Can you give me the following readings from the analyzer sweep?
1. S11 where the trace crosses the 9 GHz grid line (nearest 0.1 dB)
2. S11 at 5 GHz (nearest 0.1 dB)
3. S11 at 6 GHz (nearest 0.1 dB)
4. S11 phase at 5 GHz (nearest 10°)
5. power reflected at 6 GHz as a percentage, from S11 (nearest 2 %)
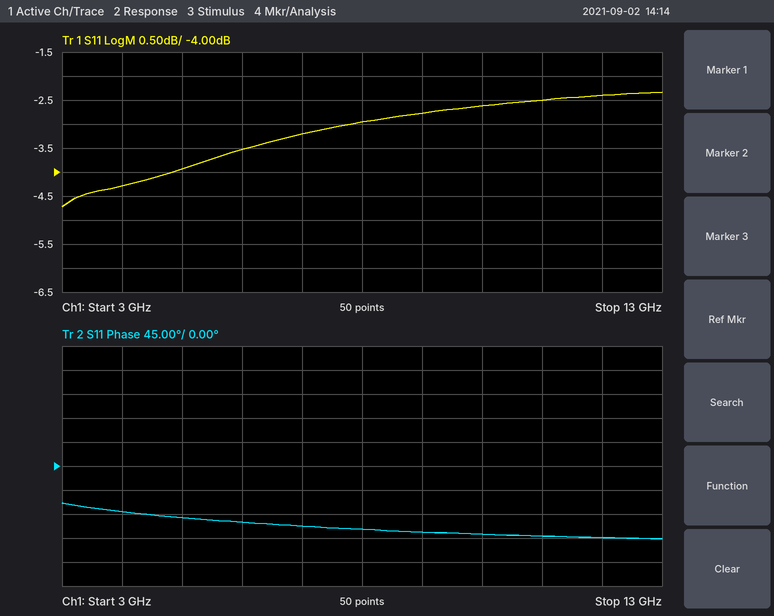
-2.8 dB
-3.9 dB
-3.5 dB
-100°
44 %
